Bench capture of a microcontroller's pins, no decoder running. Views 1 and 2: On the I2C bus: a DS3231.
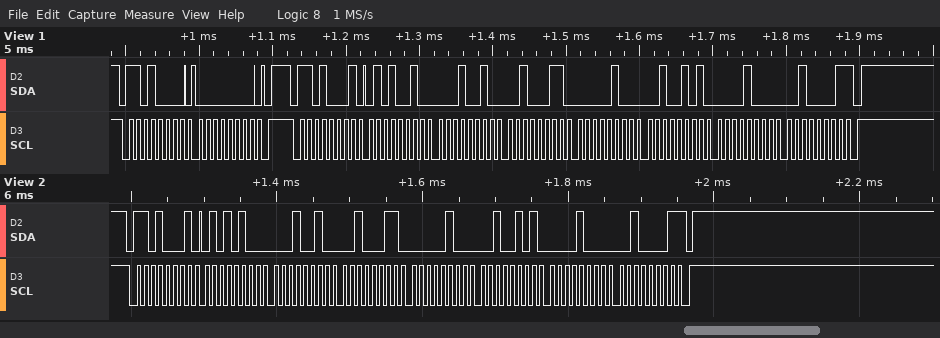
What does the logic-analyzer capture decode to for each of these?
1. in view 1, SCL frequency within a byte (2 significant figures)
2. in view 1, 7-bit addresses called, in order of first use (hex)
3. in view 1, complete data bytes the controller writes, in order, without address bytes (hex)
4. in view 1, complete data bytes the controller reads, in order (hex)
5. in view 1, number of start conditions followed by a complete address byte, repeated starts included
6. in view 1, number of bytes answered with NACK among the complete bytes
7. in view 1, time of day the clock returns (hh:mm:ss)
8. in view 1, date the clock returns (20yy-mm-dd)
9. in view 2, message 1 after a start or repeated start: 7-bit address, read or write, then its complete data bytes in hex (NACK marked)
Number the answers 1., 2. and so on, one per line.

1. 100 kHz
2. 0x68
3. 00
4. 52 12 23 04 25 08 21
5. 2
6. 1
7. 23:12:52
8. 2021-08-25
9. 0x68 read: 54 12 23 04 25 08 21 NACK
